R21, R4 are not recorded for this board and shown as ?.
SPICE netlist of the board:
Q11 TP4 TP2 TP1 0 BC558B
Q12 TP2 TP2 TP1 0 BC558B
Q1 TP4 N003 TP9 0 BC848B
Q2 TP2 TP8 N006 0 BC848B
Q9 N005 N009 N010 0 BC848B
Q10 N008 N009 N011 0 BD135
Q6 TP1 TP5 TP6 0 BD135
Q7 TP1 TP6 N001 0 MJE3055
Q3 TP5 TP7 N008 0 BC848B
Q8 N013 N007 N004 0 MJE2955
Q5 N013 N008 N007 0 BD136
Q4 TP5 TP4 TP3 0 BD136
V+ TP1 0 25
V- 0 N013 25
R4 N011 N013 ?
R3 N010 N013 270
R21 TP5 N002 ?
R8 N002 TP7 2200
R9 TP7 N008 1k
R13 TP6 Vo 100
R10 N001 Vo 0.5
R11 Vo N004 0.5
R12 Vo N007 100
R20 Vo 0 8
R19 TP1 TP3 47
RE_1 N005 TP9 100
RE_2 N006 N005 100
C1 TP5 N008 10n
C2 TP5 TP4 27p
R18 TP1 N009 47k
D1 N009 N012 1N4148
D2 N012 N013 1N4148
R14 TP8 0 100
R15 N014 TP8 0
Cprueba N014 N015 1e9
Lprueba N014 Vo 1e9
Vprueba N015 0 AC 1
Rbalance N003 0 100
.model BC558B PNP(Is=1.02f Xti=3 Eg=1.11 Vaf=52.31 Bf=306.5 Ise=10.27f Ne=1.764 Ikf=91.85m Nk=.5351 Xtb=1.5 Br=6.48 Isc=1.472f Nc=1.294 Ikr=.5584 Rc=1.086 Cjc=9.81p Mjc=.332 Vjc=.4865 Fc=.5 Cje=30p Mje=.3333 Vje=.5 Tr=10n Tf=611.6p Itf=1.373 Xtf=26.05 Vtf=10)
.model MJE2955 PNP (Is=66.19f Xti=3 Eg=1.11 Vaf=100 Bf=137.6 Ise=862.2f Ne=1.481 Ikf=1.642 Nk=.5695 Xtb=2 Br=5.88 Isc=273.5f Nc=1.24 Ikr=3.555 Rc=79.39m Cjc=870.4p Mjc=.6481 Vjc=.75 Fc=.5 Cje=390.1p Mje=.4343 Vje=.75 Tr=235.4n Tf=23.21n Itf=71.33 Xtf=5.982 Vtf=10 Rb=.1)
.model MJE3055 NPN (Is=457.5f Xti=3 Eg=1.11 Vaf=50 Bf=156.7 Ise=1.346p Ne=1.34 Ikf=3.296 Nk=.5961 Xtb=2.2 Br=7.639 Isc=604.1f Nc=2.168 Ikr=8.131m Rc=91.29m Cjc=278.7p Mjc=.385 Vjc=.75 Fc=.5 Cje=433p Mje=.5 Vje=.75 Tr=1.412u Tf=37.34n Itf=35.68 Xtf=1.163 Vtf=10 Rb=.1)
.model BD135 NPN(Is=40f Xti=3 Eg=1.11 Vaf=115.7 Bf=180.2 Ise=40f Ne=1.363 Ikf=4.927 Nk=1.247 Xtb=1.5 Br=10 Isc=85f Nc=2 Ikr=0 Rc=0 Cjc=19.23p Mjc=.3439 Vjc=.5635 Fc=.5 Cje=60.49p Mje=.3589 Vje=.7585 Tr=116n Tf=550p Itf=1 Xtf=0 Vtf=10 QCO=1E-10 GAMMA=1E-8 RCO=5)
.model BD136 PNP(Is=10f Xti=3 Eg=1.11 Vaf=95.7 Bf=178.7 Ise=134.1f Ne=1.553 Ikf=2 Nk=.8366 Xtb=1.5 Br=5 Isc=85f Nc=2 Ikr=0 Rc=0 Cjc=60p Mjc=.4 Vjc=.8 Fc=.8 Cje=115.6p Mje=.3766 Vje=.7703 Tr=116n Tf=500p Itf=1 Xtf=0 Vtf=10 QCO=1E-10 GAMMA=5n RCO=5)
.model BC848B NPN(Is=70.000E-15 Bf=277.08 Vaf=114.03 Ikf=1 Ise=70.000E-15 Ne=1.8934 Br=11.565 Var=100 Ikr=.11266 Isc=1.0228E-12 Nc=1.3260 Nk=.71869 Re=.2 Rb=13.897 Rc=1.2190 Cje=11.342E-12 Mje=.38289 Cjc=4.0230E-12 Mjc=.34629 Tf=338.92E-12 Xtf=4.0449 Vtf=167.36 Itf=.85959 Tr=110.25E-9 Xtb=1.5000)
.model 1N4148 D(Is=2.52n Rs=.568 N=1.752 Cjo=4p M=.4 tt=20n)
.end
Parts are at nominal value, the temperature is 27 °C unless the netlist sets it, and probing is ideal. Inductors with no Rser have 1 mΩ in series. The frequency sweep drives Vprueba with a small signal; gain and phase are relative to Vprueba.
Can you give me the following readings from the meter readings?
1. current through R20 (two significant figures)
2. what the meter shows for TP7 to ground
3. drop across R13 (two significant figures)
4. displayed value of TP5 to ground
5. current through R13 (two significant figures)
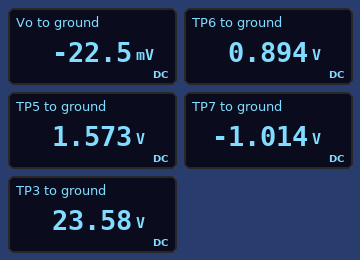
2.8 mA
-1.014 V
920 mV
1.573 V
9.2 mA
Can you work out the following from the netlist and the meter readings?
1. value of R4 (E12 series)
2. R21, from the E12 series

15 Ω
1 kΩ
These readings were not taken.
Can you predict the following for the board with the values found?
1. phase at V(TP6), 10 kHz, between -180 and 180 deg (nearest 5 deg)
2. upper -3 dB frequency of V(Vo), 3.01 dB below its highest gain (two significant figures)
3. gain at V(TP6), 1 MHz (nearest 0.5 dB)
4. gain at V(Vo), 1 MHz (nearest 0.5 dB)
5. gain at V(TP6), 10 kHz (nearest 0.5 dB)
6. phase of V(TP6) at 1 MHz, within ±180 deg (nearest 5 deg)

120 deg
5.4 kHz
29.0 dB
29.0 dB
68.0 dB
85 deg
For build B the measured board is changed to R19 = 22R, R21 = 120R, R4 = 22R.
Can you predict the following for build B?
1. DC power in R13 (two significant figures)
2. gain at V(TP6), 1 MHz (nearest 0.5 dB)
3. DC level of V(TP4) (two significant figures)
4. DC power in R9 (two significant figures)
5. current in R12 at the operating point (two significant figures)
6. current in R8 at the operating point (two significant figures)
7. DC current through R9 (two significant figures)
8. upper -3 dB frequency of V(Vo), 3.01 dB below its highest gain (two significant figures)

2.5 mW
29.0 dB
24 V
470 µW
6.0 mA
760 µA
690 µA
4.8 kHz
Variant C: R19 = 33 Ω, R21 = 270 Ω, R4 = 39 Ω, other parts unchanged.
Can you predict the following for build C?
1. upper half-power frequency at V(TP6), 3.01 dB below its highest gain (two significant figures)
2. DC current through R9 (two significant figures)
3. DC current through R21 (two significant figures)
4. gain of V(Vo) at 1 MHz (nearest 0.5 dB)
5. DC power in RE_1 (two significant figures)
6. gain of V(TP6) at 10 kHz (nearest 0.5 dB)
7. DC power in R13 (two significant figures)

3.6 kHz
670 µA
710 µA
18.0 dB
110 µW
68.5 dB
2.5 mW
